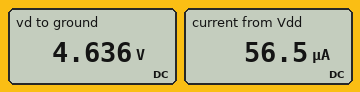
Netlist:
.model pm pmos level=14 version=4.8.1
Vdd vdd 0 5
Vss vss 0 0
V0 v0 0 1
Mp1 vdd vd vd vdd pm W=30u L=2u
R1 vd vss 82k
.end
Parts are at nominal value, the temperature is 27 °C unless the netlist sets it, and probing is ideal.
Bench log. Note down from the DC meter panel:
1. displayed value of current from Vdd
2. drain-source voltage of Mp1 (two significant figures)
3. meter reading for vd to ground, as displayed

56.5 µA
360 mV
4.636 V
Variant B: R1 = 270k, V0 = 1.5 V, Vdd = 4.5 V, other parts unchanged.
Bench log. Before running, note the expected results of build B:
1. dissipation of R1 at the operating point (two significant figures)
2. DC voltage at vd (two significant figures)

66 µW
4.2 V
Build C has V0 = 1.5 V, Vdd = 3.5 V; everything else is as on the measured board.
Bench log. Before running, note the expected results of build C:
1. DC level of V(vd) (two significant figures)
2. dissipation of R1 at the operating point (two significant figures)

3.2 V
120 µW
